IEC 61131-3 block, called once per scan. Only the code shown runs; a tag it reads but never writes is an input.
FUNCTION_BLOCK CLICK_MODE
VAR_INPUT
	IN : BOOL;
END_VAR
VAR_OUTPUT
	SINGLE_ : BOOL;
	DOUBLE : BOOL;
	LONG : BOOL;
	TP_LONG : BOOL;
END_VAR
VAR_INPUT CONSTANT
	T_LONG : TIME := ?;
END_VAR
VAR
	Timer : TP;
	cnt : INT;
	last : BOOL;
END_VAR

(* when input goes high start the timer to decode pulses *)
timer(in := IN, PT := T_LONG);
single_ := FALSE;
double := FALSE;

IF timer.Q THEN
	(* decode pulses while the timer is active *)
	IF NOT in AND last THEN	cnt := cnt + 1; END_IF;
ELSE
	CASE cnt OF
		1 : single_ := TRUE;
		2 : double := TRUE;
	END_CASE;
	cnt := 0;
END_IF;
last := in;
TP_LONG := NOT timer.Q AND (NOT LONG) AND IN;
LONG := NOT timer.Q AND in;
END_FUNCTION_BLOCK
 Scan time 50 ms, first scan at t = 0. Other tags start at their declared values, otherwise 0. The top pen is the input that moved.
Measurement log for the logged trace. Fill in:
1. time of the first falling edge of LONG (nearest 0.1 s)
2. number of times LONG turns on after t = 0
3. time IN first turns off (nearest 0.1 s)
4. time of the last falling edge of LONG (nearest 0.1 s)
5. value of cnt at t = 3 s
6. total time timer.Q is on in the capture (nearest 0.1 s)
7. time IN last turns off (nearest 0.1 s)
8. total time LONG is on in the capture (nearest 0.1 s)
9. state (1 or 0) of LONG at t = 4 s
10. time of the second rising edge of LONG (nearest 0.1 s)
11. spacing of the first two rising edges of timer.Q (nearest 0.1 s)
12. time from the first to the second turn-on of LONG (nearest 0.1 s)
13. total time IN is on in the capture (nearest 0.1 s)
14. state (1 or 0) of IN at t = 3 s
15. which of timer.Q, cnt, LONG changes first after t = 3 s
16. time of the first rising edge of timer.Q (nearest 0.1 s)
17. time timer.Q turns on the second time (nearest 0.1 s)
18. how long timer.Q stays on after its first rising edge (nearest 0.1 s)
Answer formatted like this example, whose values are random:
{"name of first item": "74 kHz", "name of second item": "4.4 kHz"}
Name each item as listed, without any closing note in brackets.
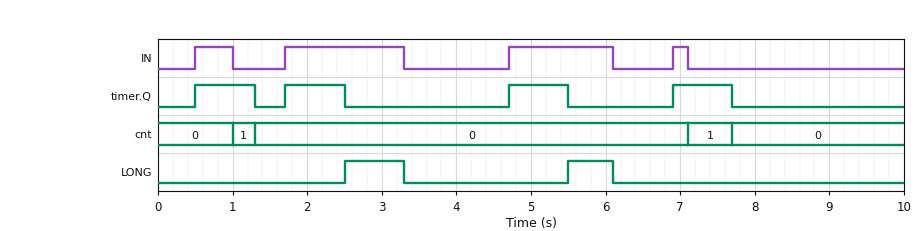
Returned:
{"time of the first falling edge of LONG": "3.3 s", "number of times LONG turns on after t = 0": "2", "time IN first turns off": "1.0 s", "time of the last falling edge of LONG": "6.1 s", "value of cnt at t = 3 s": "0", "total time timer.Q is on in the capture": "3.2 s", "time IN last turns off": "7.1 s", "total time LONG is on in the capture": "1.4 s", "state (1 or 0) of LONG at t = 4 s": "0", "time of the second rising edge of LONG": "5.5 s", "spacing of the first two rising edges of timer.Q": "1.2 s", "time from the first to the second turn-on of LONG": "3.0 s", "total time IN is on in the capture": "3.7 s", "state (1 or 0) of IN at t = 3 s": "1", "which of timer.Q, cnt, LONG changes first after t = 3 s": "LONG", "time of the first rising edge of timer.Q": "0.5 s", "time timer.Q turns on the second time": "1.7 s", "how long timer.Q stays on after its first rising edge": "0.8 s"}
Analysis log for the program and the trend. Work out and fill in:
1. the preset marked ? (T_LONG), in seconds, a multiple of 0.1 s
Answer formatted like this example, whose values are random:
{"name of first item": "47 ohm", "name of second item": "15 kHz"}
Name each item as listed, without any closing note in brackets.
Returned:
{"the preset marked ? (T_LONG), in seconds, a multiple of 0.1 s": "0.8 s"}
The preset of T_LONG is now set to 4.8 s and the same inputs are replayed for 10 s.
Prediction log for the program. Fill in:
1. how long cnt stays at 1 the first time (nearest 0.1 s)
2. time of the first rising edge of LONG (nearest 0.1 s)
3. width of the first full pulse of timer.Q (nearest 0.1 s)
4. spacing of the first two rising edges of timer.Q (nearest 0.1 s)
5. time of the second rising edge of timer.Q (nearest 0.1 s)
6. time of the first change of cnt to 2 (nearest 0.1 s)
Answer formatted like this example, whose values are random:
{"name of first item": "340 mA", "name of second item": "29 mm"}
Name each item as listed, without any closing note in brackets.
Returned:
{"how long cnt stays at 1 the first time": "2.3 s", "time of the first rising edge of LONG": "5.3 s", "width of the first full pulse of timer.Q": "4.8 s", "spacing of the first two rising edges of timer.Q": "6.4 s", "time of the second rising edge of timer.Q": "6.9 s", "time of the first change of cnt to 2": "3.3 s"}
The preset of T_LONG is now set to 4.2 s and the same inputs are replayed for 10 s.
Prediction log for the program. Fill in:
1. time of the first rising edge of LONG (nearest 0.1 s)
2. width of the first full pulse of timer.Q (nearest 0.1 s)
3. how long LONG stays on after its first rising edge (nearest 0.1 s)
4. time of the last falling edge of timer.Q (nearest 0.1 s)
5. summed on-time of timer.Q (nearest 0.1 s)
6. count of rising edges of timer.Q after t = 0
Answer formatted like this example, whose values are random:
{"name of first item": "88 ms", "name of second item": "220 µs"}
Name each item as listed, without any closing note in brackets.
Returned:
{"time of the first rising edge of LONG": "4.7 s", "width of the first full pulse of timer.Q": "4.2 s", "how long LONG stays on after its first rising edge": "1.4 s", "time of the last falling edge of timer.Q": "4.7 s", "summed on-time of timer.Q": "7.3 s", "count of rising edges of timer.Q after t = 0": "2"}
